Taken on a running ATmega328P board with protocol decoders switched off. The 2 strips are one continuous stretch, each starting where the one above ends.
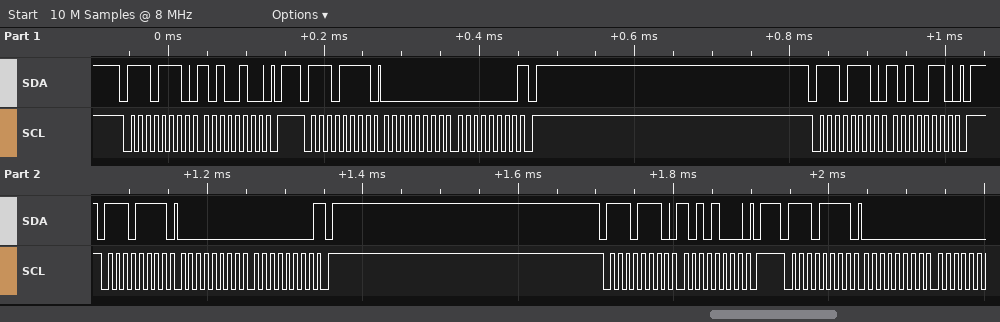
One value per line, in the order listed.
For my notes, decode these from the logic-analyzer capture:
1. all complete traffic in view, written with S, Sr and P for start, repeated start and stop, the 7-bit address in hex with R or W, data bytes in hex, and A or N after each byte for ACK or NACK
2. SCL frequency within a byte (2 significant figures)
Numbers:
S 77W A A4 A P S 77R A 00 A 00 N P S 77W A A6 A P S 77R A 00 A 00 N P S 77W A A8 A P S 77R A 00 A
100 kHz
